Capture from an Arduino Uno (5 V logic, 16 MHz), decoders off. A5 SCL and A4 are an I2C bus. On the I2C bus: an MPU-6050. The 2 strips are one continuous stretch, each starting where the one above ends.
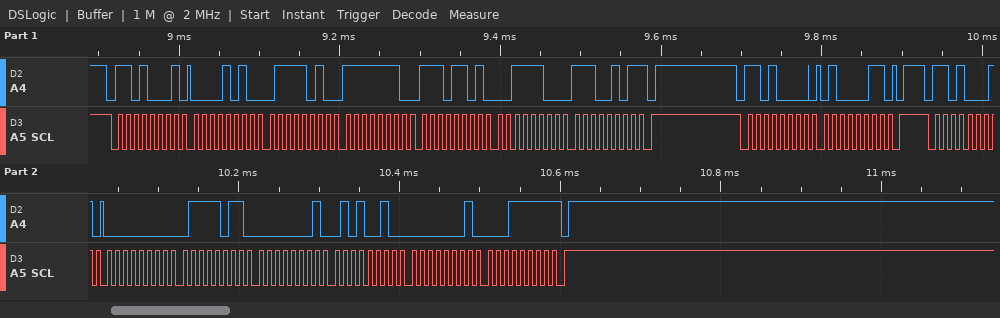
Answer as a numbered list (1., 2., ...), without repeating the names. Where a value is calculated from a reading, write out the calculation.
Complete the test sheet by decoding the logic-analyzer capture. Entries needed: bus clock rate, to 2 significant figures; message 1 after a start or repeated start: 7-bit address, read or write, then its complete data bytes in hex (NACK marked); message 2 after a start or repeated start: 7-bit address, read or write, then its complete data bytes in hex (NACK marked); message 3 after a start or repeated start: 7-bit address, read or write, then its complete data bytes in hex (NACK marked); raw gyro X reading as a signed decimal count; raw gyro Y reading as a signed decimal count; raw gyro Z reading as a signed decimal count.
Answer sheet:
1. 100 kHz
2. 0x68 read: 0A 7A FE ED 3C E5 NACK
3. 0x68 write: 43
4. 0x68 read: 00 7B 01 52 01 1F NACK
5. 0x007B = 123
6. 0x0152 = 338
7. 0x011F = 287
